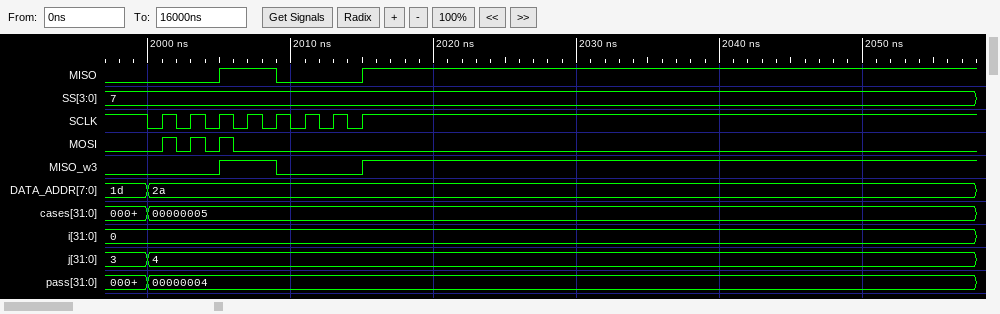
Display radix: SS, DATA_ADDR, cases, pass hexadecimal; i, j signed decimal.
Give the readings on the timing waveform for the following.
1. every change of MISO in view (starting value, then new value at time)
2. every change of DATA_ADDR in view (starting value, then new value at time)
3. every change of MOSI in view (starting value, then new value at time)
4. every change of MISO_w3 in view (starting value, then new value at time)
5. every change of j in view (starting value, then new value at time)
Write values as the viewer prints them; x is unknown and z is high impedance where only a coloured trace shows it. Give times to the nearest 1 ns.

0, 1 at 2005 ns, 0 at 2009 ns, 1 at 2015 ns
1d, 2a at 2000 ns
0, 1 at 2001 ns, 0 at 2002 ns, 1 at 2003 ns, 0 at 2004 ns, 1 at 2005 ns, 0 at 2006 ns
0, 1 at 2005 ns, 0 at 2009 ns, 1 at 2015 ns
3, 4 at 2000 ns
